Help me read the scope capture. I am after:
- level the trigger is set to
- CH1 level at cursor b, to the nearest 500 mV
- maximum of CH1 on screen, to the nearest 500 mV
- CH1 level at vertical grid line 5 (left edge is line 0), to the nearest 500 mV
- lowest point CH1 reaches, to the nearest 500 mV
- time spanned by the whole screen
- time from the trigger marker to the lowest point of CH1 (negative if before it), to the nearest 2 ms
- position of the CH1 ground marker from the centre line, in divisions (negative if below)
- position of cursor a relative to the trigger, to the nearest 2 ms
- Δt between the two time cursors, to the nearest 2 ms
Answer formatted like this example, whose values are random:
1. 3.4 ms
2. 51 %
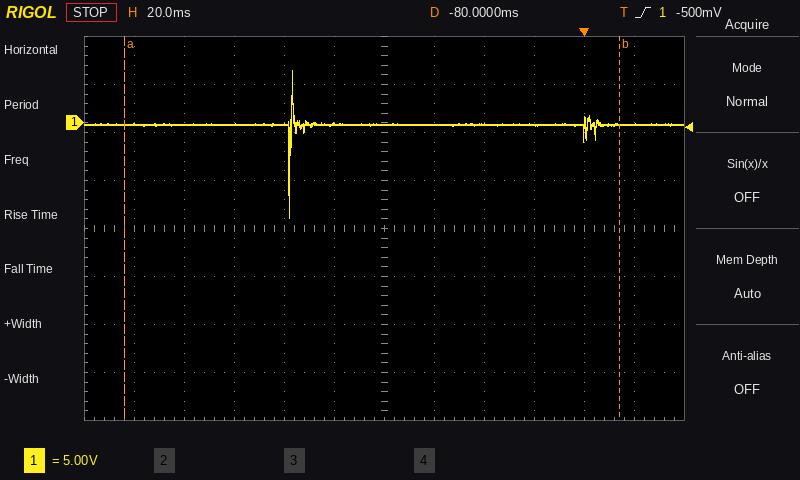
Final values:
1. -500 mV
2. 0.0 V
3. 5.5 V
4. 0.0 V
5. -10.0 V
6. 240 ms
7. -118 ms
8. +2.2 div
9. -184 ms
10. 198 ms
